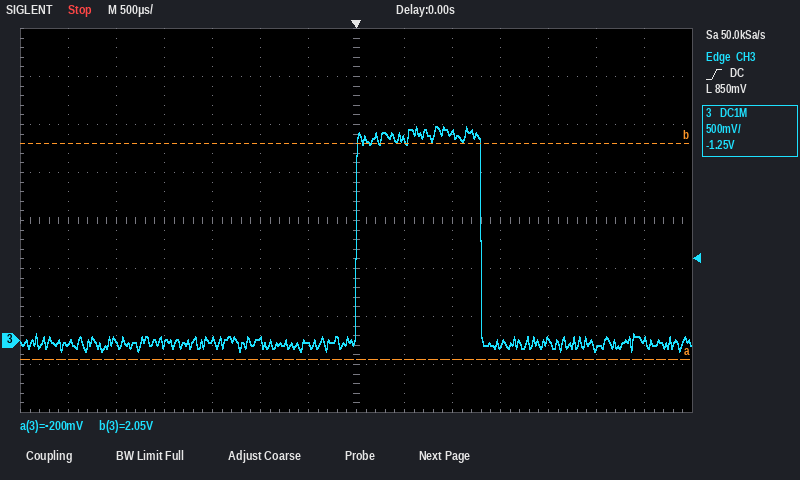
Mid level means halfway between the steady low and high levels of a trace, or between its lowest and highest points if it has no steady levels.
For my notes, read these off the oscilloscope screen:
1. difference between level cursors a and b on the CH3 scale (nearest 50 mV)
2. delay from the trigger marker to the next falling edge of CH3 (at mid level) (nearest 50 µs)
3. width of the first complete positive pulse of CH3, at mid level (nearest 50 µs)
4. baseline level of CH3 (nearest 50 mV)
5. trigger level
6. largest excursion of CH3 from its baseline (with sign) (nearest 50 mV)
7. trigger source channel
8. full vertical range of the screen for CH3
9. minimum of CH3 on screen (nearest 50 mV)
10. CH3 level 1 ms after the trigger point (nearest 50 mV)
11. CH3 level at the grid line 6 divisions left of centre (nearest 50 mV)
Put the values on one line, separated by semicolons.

2.25 V; 1.30 ms; 1.30 ms; -50 mV; 850 mV; +2.25 V; CH3; 4 V; -100 mV; 2.15 V; -50 mV
